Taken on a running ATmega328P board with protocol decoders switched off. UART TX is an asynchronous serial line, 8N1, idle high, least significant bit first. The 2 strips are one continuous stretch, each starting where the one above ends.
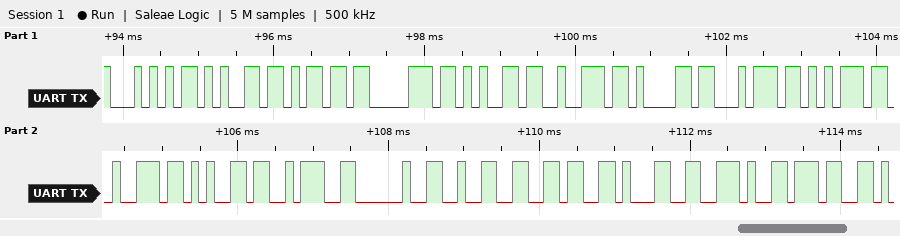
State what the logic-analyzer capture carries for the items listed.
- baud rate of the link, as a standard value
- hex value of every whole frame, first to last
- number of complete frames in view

9600 baud
54 65 6D 70 65 72 61 74 75 72 65 3A 20 32 36 31 2E 37
18
